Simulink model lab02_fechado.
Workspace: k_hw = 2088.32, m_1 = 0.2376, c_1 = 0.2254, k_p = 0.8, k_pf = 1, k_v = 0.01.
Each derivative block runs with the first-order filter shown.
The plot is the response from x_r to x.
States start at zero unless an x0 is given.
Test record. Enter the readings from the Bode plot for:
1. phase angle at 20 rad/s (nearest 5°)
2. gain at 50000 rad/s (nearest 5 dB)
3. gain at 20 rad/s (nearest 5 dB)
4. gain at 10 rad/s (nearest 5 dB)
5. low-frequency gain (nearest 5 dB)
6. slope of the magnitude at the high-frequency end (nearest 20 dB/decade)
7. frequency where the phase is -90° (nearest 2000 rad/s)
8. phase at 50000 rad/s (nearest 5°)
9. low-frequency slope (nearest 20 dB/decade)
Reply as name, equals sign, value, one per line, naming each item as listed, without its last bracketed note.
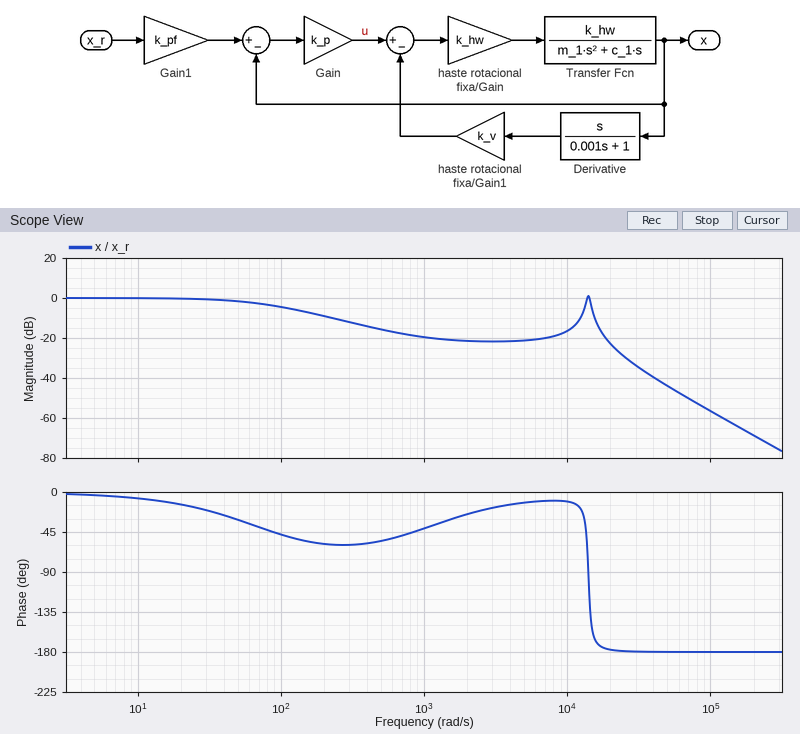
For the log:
phase angle at 20 rad/s = -15°
gain at 50000 rad/s = -45 dB
gain at 20 rad/s = 0 dB
gain at 10 rad/s = 0 dB
low-frequency gain = 0 dB
slope of the magnitude at the high-frequency end = -40 dB/decade
frequency where the phase is -90° = 14000 rad/s
phase at 50000 rad/s = -180°
low-frequency slope = 0 dB/decade
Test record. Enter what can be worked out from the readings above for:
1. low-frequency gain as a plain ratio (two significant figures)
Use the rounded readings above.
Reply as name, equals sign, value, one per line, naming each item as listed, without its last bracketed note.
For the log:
low-frequency gain as a plain ratio = 1.0
